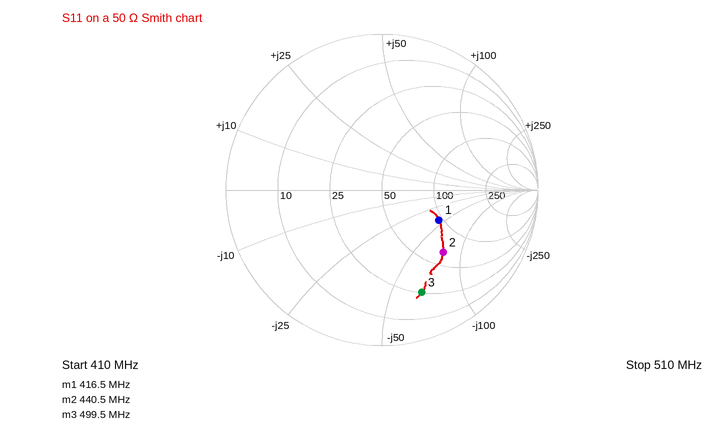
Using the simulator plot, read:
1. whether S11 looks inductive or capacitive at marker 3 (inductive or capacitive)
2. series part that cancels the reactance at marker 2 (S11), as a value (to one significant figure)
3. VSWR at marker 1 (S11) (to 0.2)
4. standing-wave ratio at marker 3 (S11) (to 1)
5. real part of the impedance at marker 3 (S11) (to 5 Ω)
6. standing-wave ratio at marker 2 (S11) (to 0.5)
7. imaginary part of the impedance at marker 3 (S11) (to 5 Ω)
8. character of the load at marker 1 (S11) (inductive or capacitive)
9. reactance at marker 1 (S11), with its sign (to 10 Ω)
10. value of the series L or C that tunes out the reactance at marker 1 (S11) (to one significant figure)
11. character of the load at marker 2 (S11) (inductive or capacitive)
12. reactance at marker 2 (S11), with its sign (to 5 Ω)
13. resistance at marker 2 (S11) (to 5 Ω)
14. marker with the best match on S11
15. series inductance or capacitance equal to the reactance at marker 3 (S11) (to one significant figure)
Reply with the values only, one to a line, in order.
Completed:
capacitive
30 nH
2.4
6
25 Ω
3.5
-65 Ω
capacitive
-40 Ω
20 nH
capacitive
-75 Ω
65 Ω
marker 1
5 pF
